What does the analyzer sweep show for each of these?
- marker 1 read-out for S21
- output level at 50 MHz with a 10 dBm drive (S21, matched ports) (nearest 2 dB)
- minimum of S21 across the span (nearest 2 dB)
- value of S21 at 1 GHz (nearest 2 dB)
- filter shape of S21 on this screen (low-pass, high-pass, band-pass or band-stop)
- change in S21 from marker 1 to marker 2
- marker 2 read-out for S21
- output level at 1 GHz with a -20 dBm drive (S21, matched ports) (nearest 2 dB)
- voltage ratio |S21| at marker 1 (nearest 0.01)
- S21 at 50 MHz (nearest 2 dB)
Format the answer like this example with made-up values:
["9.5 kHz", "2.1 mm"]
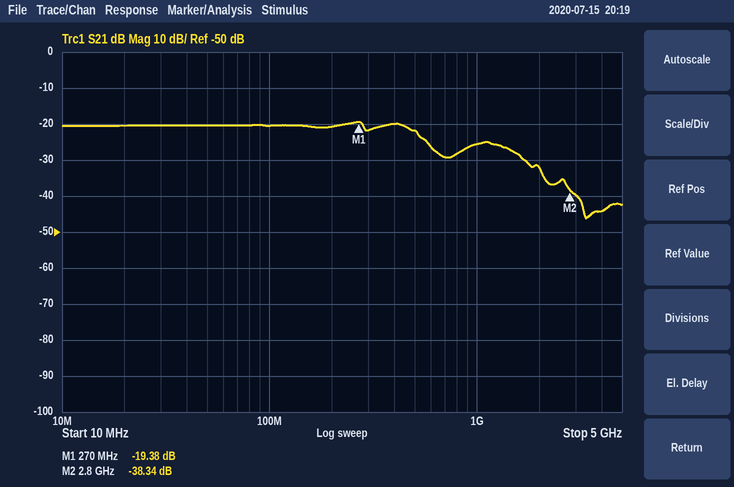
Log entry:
["-19.38 dB", "-10 dBm", "-46 dB", "-26 dB", "low-pass", "-18.96 dB", "-38.34 dB", "-46 dBm", "0.11", "-20 dB"]
